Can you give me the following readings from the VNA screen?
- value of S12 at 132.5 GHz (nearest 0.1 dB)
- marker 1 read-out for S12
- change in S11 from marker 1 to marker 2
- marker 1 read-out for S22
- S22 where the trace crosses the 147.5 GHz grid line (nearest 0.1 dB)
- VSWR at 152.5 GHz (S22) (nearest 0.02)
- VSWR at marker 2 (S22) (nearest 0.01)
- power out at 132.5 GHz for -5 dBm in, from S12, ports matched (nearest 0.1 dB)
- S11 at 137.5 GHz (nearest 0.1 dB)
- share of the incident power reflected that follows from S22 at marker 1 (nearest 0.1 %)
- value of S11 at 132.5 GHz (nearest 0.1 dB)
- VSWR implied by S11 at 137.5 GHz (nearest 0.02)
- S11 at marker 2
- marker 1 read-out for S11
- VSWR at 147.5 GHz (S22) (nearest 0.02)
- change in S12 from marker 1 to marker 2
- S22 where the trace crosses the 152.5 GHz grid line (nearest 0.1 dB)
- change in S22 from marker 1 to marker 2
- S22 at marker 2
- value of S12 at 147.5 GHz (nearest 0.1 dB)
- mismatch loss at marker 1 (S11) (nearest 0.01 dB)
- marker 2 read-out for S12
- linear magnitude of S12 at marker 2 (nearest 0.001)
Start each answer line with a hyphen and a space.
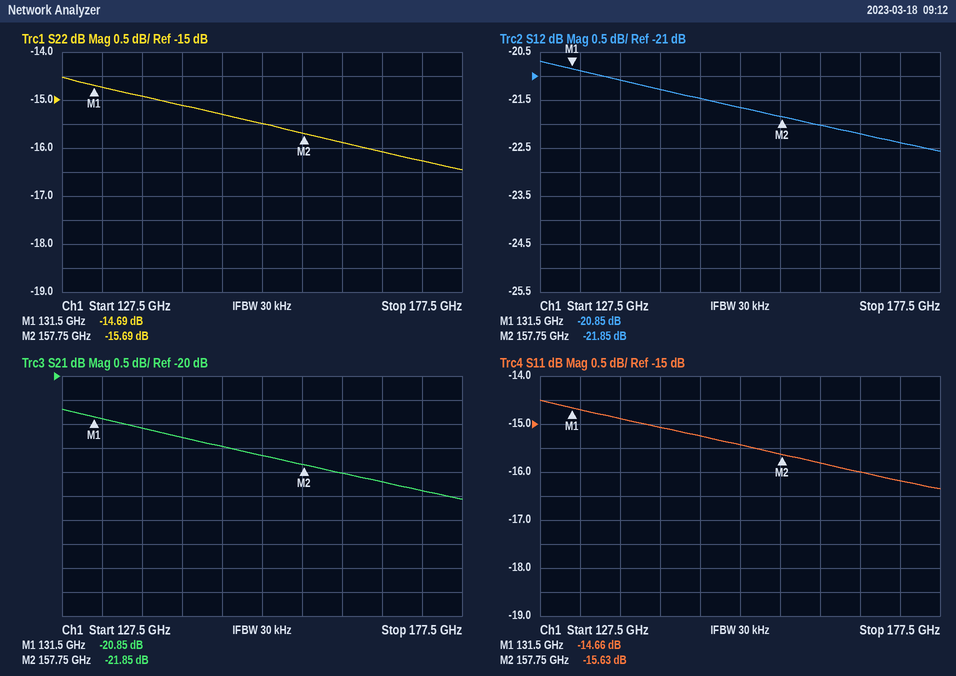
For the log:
- -20.9 dB
- -20.85 dB
- -0.97 dB
- -14.69 dB
- -15.3 dB
- 1.40
- 1.39
- -25.9 dBm
- -14.9 dB
- 3.4 %
- -14.7 dB
- 1.44
- -15.63 dB
- -14.66 dB
- 1.42
- -1.00 dB
- -15.5 dB
- -1.00 dB
- -15.69 dB
- -21.5 dB
- 0.15 dB
- -21.85 dB
- 0.081
